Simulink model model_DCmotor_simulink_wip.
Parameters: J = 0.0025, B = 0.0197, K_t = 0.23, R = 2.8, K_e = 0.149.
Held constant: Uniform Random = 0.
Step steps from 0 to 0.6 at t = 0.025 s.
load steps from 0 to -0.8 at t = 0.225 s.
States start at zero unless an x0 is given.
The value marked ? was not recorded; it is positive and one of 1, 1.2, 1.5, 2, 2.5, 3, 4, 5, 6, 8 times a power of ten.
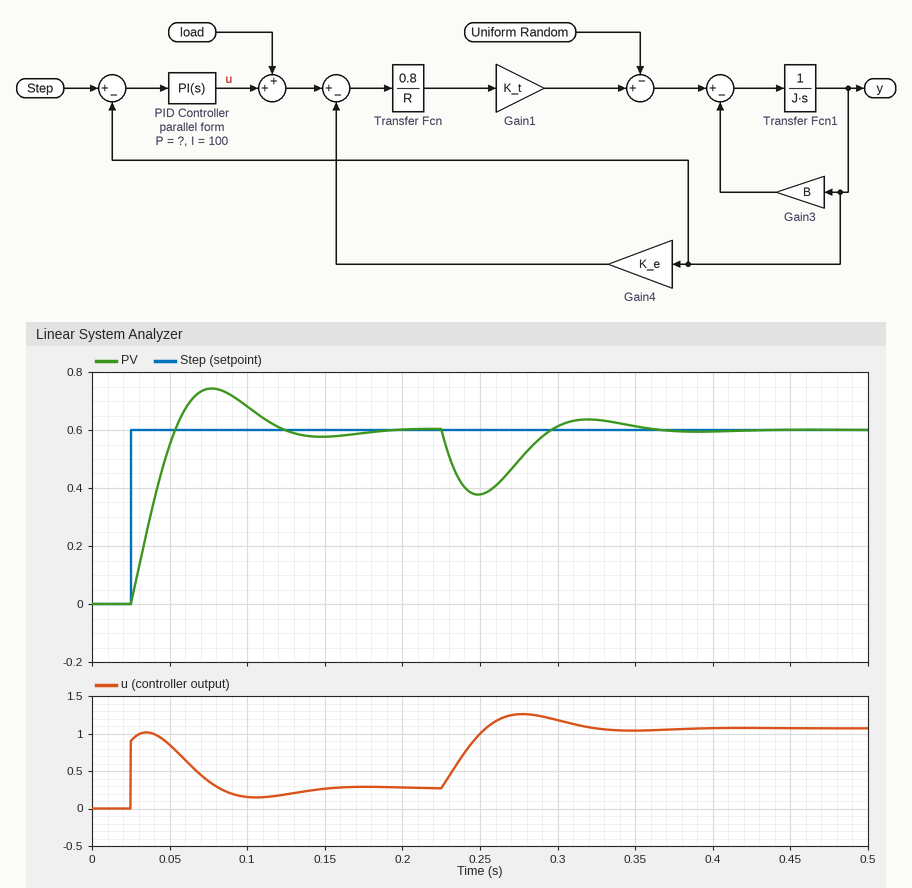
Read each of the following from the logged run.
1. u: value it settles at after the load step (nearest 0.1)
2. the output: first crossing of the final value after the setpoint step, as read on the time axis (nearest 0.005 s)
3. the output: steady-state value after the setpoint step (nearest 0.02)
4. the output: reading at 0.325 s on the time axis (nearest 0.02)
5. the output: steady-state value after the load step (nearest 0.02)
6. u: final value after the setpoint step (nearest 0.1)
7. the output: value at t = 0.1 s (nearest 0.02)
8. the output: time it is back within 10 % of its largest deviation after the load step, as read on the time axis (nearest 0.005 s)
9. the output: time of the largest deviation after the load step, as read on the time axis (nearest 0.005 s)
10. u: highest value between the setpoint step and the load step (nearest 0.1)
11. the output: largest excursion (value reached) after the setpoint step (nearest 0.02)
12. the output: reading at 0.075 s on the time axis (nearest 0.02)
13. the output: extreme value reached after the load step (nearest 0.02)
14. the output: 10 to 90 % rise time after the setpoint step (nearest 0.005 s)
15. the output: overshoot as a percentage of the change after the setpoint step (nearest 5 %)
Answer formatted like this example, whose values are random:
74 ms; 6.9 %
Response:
1.1; 0.055 s; 0.60; 0.64; 0.60; 0.3; 0.68; 0.340 s; 0.250 s; 1.0; 0.74; 0.74; 0.38; 0.020 s; 25 %
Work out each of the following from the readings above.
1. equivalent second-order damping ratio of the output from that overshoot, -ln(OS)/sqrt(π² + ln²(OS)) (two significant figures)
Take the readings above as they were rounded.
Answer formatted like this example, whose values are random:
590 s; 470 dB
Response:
0.40
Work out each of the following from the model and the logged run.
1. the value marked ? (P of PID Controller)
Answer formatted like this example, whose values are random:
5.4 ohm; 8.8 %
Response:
1.5
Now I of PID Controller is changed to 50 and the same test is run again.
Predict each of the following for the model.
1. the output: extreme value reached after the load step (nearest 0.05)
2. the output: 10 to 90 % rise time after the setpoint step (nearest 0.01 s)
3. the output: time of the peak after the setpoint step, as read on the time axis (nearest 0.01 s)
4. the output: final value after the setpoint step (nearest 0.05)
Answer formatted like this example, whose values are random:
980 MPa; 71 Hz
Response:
0.35; 0.03 s; 0.10 s; 0.60
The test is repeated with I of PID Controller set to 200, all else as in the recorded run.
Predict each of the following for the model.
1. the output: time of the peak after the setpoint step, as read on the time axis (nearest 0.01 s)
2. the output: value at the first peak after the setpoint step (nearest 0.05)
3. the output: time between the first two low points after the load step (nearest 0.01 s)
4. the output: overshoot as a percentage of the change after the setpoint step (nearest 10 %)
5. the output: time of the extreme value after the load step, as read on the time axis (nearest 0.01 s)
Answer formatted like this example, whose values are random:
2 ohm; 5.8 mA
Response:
0.06 s; 0.80; 0.09 s; 40 %; 0.24 s
